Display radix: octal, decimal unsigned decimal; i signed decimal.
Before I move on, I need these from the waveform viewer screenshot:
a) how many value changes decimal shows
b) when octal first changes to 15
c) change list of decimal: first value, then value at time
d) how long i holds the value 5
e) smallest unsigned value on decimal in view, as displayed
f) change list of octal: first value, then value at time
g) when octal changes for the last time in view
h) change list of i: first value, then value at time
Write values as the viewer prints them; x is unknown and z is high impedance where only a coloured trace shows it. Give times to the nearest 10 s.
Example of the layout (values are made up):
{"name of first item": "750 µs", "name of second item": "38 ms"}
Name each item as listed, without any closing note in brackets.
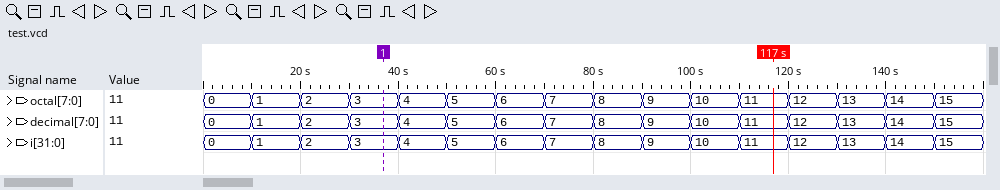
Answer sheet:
{"how many value changes decimal shows": "15", "when octal first changes to 15": "150 s", "change list of decimal: first value, then value at time": "0, 1 at 10 s, 2 at 20 s, 3 at 30 s, 4 at 40 s, 5 at 50 s, 6 at 60 s, 7 at 70 s, 8 at 80 s, 9 at 90 s, 10 at 100 s, 11 at 110 s, 12 at 120 s, 13 at 130 s, 14 at 140 s, 15 at 150 s", "how long i holds the value 5": "10 s", "smallest unsigned value on decimal in view, as displayed": "0", "change list of octal: first value, then value at time": "0, 1 at 10 s, 2 at 20 s, 3 at 30 s, 4 at 40 s, 5 at 50 s, 6 at 60 s, 7 at 70 s, 8 at 80 s, 9 at 90 s, 10 at 100 s, 11 at 110 s, 12 at 120 s, 13 at 130 s, 14 at 140 s, 15 at 150 s", "when octal changes for the last time in view": "150 s", "change list of i: first value, then value at time": "0, 1 at 10 s, 2 at 20 s, 3 at 30 s, 4 at 40 s, 5 at 50 s, 6 at 60 s, 7 at 70 s, 8 at 80 s, 9 at 90 s, 10 at 100 s, 11 at 110 s, 12 at 120 s, 13 at 130 s, 14 at 140 s, 15 at 150 s"}
